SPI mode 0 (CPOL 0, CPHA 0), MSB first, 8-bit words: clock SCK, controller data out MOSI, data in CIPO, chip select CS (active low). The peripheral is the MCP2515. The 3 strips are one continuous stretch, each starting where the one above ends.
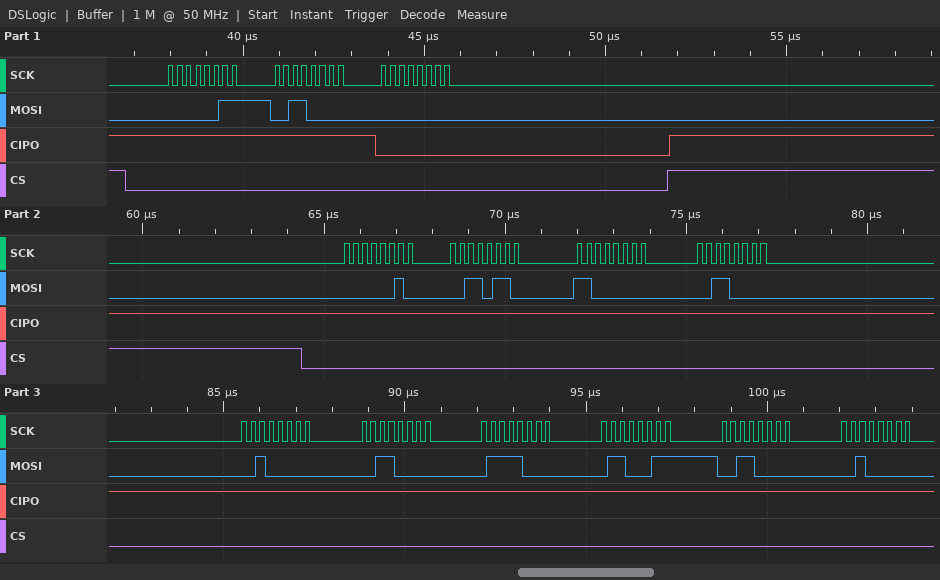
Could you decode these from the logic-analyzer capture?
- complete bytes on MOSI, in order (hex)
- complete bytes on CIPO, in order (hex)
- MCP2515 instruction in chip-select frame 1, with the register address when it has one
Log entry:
03 30 00 02 36 C0 30 20 30 78 63 30 20
FF FF 00 FF FF FF FF FF FF FF FF FF FF
READ 0x30
